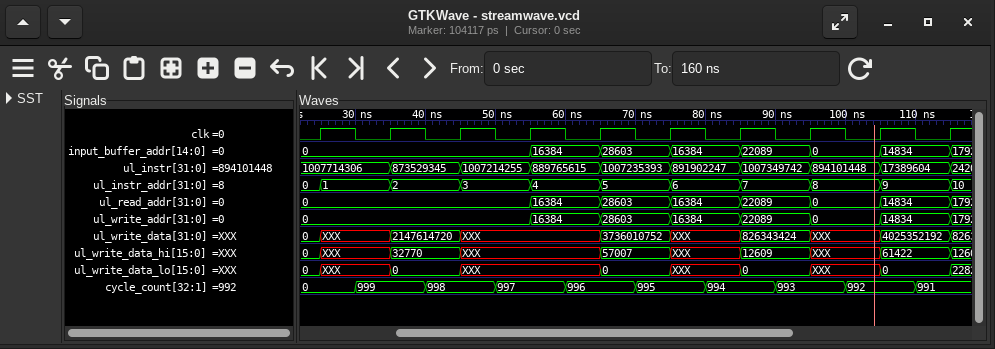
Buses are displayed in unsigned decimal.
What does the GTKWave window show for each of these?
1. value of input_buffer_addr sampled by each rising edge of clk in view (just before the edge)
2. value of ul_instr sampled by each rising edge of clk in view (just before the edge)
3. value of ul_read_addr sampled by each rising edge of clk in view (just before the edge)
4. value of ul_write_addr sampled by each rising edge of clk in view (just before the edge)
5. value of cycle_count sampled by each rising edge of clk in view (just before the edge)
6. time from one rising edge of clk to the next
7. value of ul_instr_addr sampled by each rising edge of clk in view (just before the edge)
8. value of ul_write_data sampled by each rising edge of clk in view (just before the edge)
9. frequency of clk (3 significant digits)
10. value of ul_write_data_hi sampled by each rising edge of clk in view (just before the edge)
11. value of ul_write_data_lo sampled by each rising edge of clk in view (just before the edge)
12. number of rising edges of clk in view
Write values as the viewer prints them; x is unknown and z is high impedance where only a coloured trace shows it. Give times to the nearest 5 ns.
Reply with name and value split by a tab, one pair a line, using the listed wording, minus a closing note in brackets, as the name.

value of input_buffer_addr sampled by each rising edge of clk in view	0, 0, 0, 0, 16384, 28603, 16384, 22089, 0, 14834
value of ul_instr sampled by each rising edge of clk in view	1007714306, 1007714306, 873529345, 1007214255, 889765615, 1007235393, 891902247, 1007349742, 894101448, 17389604
value of ul_read_addr sampled by each rising edge of clk in view	0, 0, 0, 0, 16384, 28603, 16384, 22089, 0, 14834
value of ul_write_addr sampled by each rising edge of clk in view	0, 0, 0, 0, 16384, 28603, 16384, 22089, 0, 14834
value of cycle_count sampled by each rising edge of clk in view	0, 999, 998, 997, 996, 995, 994, 993, 992, 991
time from one rising edge of clk to the next	10 ns
value of ul_instr_addr sampled by each rising edge of clk in view	0, 1, 2, 3, 4, 5, 6, 7, 8, 9
value of ul_write_data sampled by each rising edge of clk in view	0, XXX, 2147614720, XXX, XXX, 3736010752, XXX, 826343424, XXX, 4025352192
frequency of clk	100 MHz
value of ul_write_data_hi sampled by each rising edge of clk in view	0, XXX, 32770, XXX, XXX, 57007, XXX, 12609, XXX, 61422
value of ul_write_data_lo sampled by each rising edge of clk in view	0, XXX, 0, XXX, XXX, 0, XXX, 0, XXX, 0
number of rising edges of clk in view	10
